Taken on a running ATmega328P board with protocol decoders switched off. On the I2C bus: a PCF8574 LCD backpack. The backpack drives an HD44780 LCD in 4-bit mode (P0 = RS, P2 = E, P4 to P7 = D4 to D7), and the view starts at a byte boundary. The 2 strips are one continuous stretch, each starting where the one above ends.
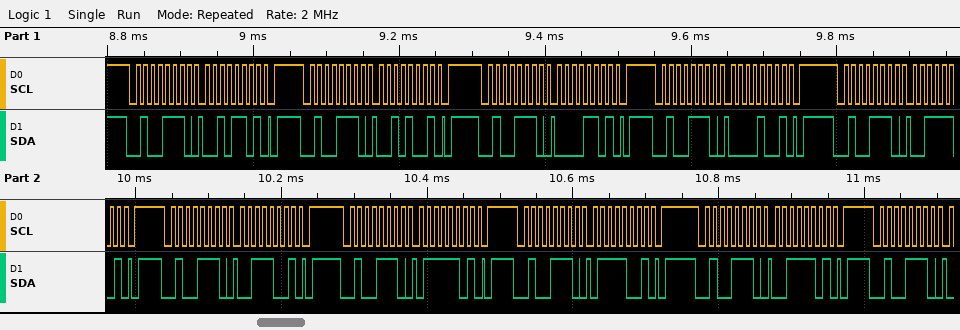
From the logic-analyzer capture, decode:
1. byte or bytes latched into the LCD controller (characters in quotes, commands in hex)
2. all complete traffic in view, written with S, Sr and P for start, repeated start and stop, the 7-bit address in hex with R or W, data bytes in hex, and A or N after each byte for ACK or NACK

' ' '7'
S 27W A 2D A P S 27W A 29 A P S 27W A 0D A P S 27W A 09 A P S 27W A 3D A P S 27W A 39 A P S 27W A 7D A P S 27W A 79 A P S 27W A 3D A P S 27W A
